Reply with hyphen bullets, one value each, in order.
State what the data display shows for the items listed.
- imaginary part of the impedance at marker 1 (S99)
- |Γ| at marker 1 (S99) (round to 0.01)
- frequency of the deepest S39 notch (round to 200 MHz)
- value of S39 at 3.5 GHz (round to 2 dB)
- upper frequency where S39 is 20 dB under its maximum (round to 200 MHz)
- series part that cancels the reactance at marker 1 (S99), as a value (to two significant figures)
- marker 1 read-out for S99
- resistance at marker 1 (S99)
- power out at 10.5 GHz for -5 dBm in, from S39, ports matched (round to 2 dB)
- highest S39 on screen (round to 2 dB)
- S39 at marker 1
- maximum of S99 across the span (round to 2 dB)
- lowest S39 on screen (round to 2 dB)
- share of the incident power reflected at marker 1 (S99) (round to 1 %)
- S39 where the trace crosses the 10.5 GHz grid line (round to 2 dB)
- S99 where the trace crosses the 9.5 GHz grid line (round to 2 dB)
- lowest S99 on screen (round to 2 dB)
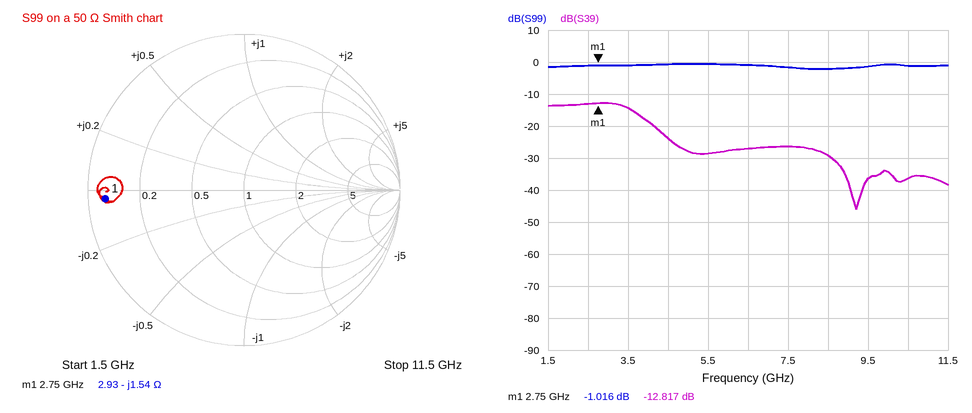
- -1.54 Ω
- 0.89
- 9.2 GHz
- -14 dB
- 8.8 GHz
- 89 pH
- -1.016 dB
- 2.93 Ω
- -42 dBm
- -12 dB
- -12.817 dB
- 0 dB
- -46 dB
- 79 %
- -36 dB
- -2 dB
- -2 dB
